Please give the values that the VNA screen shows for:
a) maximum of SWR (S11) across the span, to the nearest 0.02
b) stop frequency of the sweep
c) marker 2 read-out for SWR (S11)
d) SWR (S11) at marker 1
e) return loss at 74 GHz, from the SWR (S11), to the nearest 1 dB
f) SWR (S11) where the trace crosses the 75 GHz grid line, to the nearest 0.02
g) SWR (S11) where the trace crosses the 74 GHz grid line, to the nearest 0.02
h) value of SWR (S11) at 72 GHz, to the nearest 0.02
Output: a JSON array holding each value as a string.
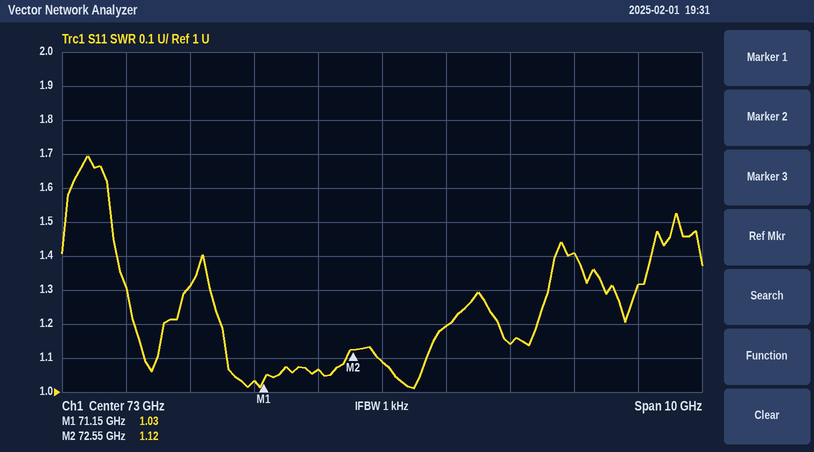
["1.70", "78 GHz", "1.12", "1.03", "21 dB", "1.14", "1.20", "1.06"]
